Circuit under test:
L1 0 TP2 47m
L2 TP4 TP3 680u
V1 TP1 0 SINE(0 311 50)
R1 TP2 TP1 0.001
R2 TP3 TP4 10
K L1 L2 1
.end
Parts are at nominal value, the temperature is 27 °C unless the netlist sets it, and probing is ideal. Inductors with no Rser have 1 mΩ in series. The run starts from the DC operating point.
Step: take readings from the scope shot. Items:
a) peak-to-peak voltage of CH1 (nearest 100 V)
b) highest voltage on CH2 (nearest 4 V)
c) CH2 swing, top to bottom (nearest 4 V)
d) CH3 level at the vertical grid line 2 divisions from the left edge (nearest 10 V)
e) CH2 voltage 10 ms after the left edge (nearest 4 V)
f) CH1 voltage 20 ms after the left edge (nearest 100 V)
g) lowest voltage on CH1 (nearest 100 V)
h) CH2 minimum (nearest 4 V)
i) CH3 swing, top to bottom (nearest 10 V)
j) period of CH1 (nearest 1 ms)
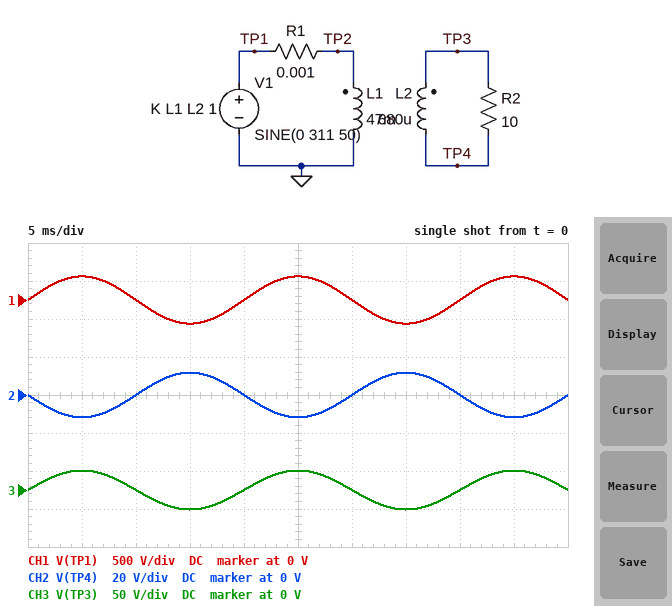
600 V
12 V
24 V
0 V
0 V
0 V
-300 V
-12 V
50 V
20 ms
